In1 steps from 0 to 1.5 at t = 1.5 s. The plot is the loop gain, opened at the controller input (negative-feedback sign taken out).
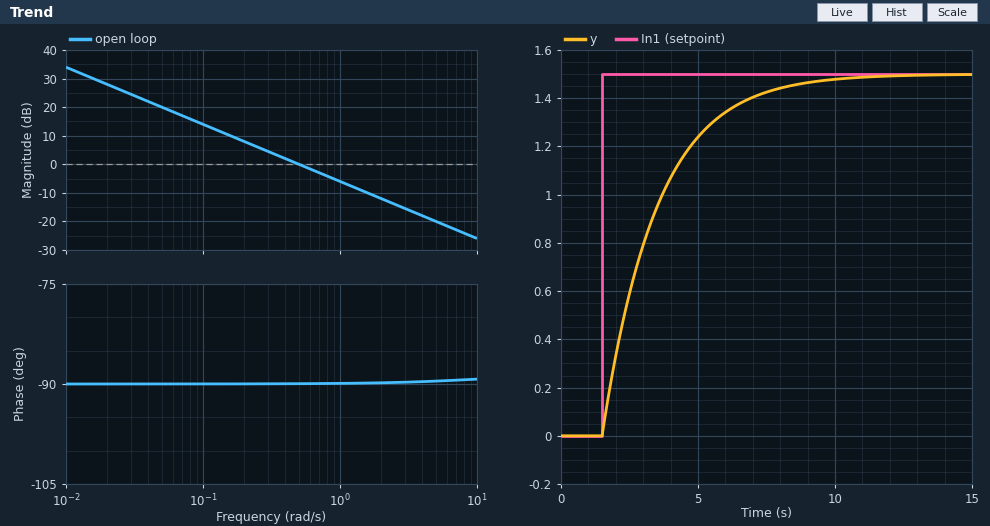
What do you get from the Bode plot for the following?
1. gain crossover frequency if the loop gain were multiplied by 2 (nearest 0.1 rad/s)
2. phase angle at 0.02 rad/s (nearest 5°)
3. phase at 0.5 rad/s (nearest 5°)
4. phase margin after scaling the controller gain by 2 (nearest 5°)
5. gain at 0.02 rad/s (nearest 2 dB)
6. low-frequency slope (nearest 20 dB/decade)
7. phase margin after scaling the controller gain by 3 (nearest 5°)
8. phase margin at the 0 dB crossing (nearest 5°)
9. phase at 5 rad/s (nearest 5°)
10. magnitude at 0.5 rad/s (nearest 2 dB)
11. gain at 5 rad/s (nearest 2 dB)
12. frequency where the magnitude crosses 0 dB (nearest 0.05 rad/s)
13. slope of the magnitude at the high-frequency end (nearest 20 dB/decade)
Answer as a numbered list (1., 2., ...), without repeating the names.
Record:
1. 1.0 rad/s
2. -90°
3. -90°
4. 90°
5. 28 dB
6. -20 dB/decade
7. 90°
8. 90°
9. -90°
10. 0 dB
11. -20 dB
12. 0.50 rad/s
13. -20 dB/decade
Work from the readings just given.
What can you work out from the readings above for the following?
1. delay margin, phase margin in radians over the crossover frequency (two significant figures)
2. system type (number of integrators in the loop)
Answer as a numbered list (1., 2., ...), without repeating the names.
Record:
1. 3.1 s
2. 1
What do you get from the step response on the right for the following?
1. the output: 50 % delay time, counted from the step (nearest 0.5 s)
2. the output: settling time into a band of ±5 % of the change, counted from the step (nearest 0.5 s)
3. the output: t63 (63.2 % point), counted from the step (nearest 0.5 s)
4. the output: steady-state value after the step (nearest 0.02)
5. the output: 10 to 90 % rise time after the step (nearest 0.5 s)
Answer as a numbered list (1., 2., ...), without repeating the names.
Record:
1. 1.5 s
2. 6.0 s
3. 2.0 s
4. 1.50
5. 4.5 s
